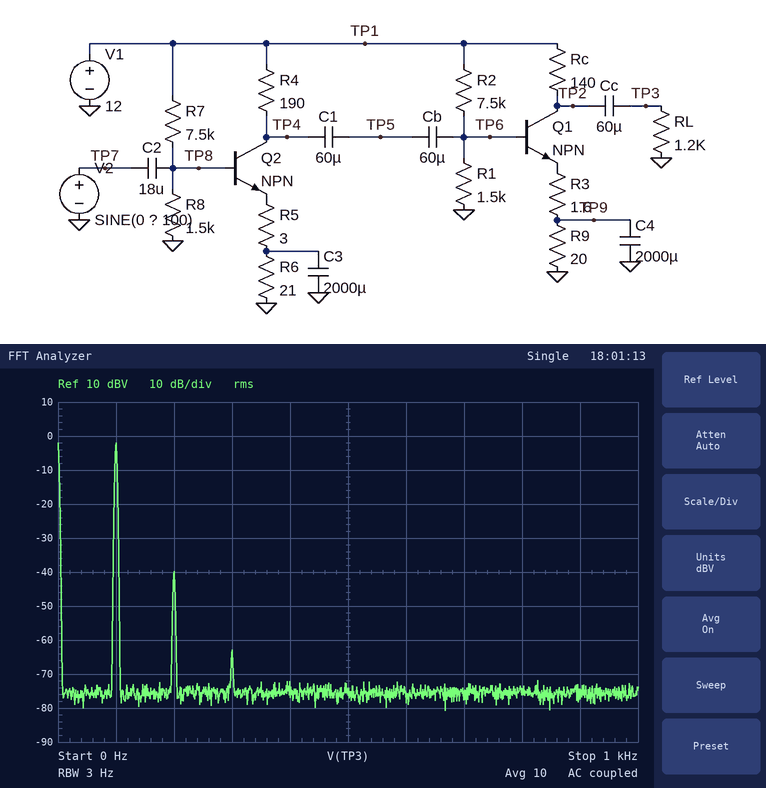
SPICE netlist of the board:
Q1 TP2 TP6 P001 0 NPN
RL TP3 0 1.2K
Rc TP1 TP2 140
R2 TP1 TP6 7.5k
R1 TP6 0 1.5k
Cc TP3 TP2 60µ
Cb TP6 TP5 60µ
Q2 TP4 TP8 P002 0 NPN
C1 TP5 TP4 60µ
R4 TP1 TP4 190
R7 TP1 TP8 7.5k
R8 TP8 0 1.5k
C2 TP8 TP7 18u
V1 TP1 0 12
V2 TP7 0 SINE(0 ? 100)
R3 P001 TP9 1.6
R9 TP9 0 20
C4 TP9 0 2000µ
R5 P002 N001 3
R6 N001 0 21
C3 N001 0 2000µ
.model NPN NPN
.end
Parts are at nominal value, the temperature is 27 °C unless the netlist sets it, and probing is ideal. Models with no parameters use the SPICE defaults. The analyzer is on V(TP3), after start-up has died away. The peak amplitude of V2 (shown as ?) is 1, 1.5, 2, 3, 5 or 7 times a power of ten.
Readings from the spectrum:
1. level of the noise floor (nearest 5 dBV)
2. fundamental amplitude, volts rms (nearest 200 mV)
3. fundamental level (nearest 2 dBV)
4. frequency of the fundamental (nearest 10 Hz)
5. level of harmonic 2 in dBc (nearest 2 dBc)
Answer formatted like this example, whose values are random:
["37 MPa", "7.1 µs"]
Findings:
["-75 dBV", "800 mV", "-2 dBV", "100 Hz", "-38 dBc"]
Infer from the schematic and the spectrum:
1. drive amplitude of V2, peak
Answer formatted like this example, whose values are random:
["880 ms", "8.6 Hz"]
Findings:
["1 mV"]
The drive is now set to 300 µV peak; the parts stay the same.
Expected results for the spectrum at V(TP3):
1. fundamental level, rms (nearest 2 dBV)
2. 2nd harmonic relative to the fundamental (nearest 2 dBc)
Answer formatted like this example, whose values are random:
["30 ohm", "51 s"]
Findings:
["-12 dBV", "-48 dBc"]
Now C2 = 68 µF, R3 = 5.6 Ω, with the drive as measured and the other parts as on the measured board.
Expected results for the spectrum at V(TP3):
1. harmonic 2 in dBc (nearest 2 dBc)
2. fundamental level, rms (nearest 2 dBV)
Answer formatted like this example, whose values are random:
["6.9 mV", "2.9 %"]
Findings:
["-48 dBc", "-8 dBV"]
